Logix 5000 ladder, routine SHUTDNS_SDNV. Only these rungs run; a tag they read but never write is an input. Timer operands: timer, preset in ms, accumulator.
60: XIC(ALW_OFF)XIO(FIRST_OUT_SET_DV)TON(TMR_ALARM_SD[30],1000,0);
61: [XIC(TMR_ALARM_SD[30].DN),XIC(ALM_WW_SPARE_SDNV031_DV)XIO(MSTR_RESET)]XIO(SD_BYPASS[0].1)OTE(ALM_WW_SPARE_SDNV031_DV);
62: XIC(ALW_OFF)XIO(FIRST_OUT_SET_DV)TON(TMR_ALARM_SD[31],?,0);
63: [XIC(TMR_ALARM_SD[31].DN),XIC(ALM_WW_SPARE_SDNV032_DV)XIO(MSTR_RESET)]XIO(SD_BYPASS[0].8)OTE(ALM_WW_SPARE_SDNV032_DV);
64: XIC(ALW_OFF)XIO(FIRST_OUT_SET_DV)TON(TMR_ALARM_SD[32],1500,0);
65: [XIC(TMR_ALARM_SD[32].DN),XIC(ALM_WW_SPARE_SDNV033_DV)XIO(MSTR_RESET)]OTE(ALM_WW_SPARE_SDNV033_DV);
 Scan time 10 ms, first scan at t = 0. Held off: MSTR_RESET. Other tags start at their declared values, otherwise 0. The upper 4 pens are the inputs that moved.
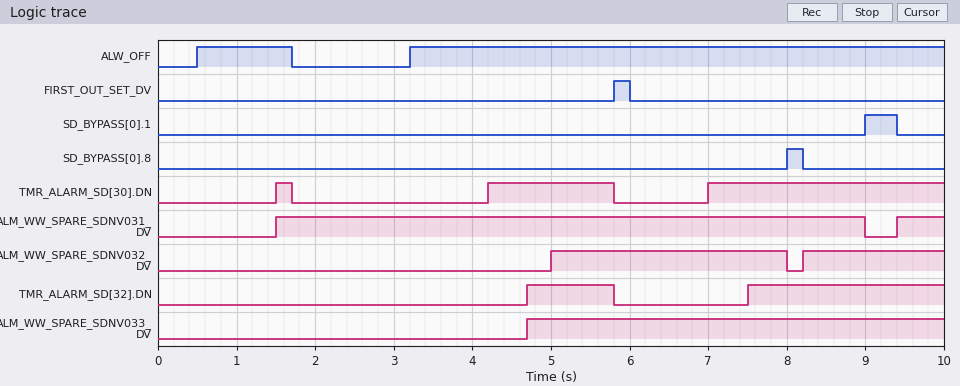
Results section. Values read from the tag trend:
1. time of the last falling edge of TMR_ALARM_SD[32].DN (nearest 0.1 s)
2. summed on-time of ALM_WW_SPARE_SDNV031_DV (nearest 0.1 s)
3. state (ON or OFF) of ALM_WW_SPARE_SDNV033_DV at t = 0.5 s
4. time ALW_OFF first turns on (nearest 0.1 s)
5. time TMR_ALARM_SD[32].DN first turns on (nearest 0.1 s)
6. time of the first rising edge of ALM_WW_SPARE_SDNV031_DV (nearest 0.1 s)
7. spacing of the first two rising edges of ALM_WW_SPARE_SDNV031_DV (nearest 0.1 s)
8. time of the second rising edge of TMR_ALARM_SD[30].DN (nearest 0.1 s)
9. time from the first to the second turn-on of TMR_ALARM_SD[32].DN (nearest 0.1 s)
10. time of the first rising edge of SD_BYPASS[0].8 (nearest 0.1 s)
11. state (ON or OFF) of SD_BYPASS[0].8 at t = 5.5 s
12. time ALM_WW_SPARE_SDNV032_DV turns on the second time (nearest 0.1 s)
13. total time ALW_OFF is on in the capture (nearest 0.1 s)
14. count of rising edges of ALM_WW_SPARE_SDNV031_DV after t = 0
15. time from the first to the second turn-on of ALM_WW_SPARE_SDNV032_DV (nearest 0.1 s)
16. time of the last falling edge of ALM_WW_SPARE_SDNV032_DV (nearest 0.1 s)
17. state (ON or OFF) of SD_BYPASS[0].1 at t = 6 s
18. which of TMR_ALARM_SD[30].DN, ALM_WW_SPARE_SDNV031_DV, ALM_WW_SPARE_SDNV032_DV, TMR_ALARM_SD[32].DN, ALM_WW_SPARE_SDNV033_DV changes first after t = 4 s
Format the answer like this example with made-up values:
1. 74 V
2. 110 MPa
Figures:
1. 5.8 s
2. 8.1 s
3. OFF
4. 0.5 s
5. 4.7 s
6. 1.5 s
7. 7.9 s
8. 4.2 s
9. 2.8 s
10. 8.0 s
11. OFF
12. 8.2 s
13. 8.0 s
14. 2
15. 3.2 s
16. 8.0 s
17. OFF
18. TMR_ALARM_SD[30].DN
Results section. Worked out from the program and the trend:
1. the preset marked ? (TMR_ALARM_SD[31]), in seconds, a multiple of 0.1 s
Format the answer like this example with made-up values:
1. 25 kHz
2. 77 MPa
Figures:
1. 1.8 s
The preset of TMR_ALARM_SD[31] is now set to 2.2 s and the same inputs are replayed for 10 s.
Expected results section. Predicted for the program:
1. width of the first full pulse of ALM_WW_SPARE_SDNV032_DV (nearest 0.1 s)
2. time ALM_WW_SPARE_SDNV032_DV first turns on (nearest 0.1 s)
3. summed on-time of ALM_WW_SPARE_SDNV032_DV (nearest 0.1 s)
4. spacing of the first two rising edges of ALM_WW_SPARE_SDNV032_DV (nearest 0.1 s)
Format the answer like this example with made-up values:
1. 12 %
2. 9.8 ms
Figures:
1. 2.6 s
2. 5.4 s
3. 4.4 s
4. 2.8 s
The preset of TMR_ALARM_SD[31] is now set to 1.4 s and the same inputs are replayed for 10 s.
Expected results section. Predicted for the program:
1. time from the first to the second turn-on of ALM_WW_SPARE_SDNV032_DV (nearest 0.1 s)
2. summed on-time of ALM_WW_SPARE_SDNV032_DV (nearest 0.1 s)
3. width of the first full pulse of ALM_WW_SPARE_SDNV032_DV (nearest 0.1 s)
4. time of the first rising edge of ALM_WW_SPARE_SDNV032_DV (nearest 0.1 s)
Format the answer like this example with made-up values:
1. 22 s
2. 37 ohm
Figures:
1. 3.6 s
2. 5.2 s
3. 3.4 s
4. 4.6 s
